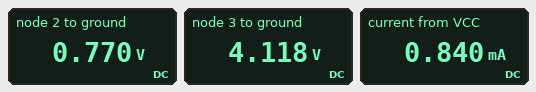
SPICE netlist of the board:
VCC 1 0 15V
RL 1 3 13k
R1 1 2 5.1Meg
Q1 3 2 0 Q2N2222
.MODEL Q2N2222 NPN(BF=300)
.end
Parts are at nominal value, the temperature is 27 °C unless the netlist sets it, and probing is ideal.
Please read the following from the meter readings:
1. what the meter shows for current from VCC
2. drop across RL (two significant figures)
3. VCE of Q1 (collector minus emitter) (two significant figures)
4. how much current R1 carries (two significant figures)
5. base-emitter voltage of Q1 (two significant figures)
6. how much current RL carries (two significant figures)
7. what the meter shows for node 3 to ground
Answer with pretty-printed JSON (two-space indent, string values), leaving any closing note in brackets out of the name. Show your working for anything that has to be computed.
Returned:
{
  "what the meter shows for current from VCC": "0.840 mA",
  "drop across RL": "15 V - 4.118 V = 11 V",
  "VCE of Q1 (collector minus emitter)": "4.118 V = 4.1 V",
  "how much current R1 carries": "(15 V - 770 mV) / 5.1 MΩ = 2.8 µA",
  "base-emitter voltage of Q1": "770 mV = 770 mV",
  "how much current RL carries": "(15 V - 4.118 V) / 13 kΩ = 840 µA",
  "what the meter shows for node 3 to ground": "4.118 V"
}
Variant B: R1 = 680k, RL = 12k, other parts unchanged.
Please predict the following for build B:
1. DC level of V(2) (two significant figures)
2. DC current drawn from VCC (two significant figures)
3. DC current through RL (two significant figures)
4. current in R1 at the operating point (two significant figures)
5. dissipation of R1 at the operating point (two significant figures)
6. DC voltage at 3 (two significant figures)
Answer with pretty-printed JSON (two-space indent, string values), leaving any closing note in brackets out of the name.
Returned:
{
  "DC level of V(2)": "780 mV",
  "DC current drawn from VCC": "1.3 mA",
  "DC current through RL": "1.2 mA",
  "current in R1 at the operating point": "21 µA",
  "dissipation of R1 at the operating point": "300 µW",
  "DC voltage at 3": "110 mV"
}
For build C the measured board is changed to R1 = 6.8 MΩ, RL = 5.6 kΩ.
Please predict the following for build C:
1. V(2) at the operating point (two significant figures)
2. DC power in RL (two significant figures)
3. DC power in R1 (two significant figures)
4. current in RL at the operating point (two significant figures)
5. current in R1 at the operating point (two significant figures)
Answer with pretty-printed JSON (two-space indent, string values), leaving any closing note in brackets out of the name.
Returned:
{
  "V(2) at the operating point": "760 mV",
  "DC power in RL": "2.2 mW",
  "DC power in R1": "30 µW",
  "current in RL at the operating point": "630 µA",
  "current in R1 at the operating point": "2.1 µA"
}
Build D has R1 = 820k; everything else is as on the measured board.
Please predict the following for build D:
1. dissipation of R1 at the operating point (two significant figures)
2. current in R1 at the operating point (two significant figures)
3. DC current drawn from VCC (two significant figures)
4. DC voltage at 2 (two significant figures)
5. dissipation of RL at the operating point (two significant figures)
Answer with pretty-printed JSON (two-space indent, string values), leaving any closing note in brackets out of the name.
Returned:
{
  "dissipation of R1 at the operating point": "250 µW",
  "current in R1 at the operating point": "17 µA",
  "DC current drawn from VCC": "1.2 mA",
  "DC voltage at 2": "780 mV",
  "dissipation of RL at the operating point": "17 mW"
}
